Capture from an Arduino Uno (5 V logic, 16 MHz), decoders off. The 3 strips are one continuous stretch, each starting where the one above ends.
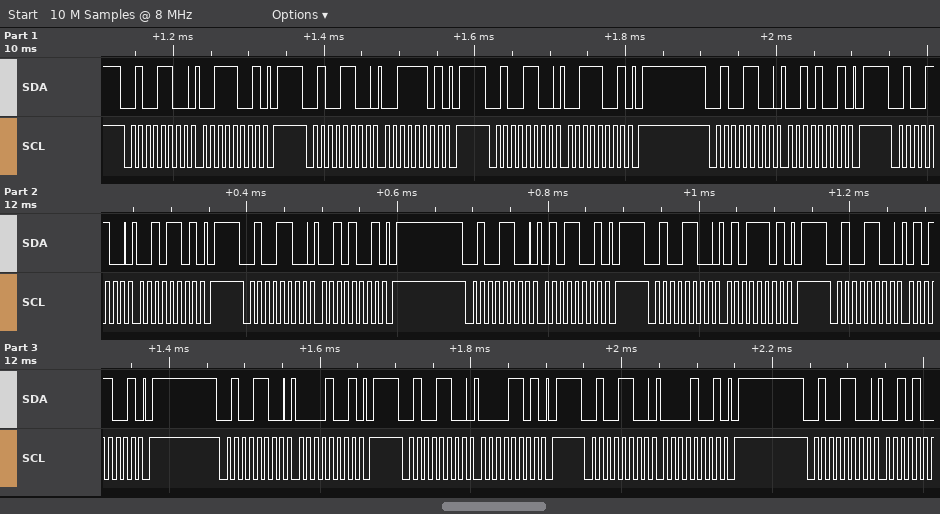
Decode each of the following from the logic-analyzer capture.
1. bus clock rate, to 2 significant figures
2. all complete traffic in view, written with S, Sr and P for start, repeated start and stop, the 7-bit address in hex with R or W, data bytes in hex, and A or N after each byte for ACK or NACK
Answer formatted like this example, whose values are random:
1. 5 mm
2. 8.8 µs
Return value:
1. 100 kHz
2. S 26W A 39 A P S 26W A 3D A P S 26W A 39 A P S 26W A 29 A P S 26W A 2D A P S 26W A 29 A P S 26W A 59 A P S 26W A 5D A P S 26W A 59 A P S 26W A 09 A P S 26W A 0D A P S 26W A 09 A P S 26W A
